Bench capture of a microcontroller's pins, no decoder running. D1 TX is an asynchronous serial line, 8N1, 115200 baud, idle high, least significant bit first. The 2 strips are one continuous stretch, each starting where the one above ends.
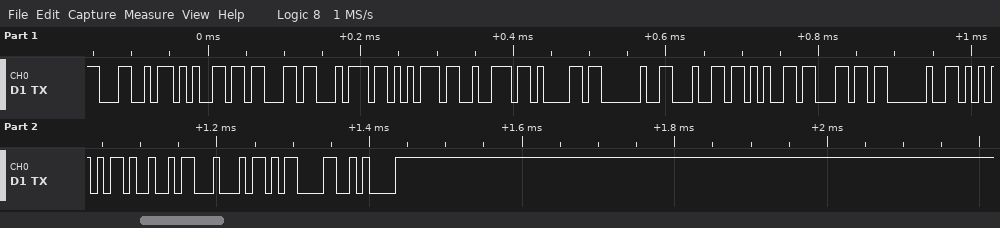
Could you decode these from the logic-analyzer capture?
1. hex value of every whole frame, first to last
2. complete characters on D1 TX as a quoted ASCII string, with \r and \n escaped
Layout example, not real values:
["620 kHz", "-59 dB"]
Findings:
["4C 65 63 74 75 72 61 20 64 65 6C 20 55 49 44 0D 0A", "\"Lectura del UID\\r\\n\""]
